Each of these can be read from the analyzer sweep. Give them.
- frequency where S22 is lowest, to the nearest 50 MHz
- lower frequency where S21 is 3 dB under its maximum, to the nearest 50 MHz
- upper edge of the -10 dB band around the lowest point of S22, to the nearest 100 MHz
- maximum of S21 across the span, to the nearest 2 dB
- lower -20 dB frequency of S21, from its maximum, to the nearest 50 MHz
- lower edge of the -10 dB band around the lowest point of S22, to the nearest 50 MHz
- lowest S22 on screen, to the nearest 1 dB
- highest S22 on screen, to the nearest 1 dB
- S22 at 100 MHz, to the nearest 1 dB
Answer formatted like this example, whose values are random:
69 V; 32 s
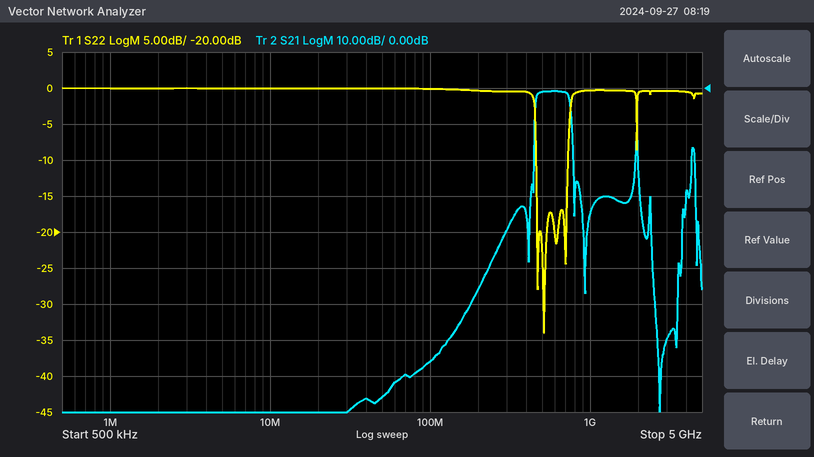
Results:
500 MHz; 450 MHz; 700 MHz; 0 dB; 450 MHz; 450 MHz; -34 dB; 0 dB; 0 dB
